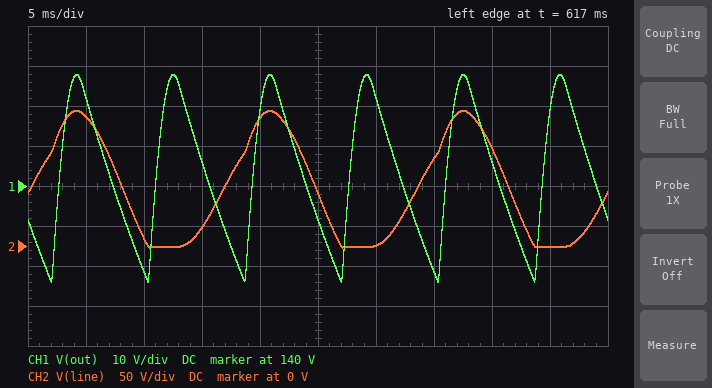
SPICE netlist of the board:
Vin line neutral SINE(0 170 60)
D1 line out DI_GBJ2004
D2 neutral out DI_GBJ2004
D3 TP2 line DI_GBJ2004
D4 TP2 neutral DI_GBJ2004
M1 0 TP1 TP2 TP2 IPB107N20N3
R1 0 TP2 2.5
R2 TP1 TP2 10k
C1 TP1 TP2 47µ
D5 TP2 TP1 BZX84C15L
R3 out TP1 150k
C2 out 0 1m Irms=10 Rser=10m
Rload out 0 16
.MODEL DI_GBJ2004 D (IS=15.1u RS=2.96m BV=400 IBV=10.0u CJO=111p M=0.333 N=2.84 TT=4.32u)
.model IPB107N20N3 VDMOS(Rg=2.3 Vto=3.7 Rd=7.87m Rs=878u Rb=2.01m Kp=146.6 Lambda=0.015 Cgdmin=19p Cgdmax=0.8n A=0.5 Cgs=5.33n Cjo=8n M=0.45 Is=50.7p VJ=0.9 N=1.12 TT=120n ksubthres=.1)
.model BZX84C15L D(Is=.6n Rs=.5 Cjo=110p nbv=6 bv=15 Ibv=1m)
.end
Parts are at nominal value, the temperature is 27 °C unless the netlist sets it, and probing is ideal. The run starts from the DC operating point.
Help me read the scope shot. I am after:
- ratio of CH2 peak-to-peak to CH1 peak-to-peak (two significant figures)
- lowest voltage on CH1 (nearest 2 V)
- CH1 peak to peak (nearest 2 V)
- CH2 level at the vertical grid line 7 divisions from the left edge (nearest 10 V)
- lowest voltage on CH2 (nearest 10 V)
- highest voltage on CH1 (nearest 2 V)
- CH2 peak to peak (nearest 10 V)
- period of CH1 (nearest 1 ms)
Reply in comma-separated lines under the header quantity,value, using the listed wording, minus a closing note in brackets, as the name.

quantity,value
ratio of CH2 peak-to-peak to CH1 peak-to-peak,3.3
lowest voltage on CH1,116 V
CH1 peak to peak,52 V
CH2 level at the vertical grid line 7 divisions from the left edge,110 V
lowest voltage on CH2,0 V
highest voltage on CH1,168 V
CH2 peak to peak,170 V
period of CH1,8 ms
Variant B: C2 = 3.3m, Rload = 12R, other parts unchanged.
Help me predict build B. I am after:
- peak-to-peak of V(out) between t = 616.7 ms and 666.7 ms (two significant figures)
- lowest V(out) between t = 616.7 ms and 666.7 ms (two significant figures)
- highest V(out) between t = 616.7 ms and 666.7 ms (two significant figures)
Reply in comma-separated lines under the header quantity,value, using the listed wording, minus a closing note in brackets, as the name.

quantity,value
peak-to-peak of V(out) between t = 616.7 ms and 666.7 ms,26 V
lowest V(out) between t = 616.7 ms and 666.7 ms,140 V
highest V(out) between t = 616.7 ms and 666.7 ms,170 V
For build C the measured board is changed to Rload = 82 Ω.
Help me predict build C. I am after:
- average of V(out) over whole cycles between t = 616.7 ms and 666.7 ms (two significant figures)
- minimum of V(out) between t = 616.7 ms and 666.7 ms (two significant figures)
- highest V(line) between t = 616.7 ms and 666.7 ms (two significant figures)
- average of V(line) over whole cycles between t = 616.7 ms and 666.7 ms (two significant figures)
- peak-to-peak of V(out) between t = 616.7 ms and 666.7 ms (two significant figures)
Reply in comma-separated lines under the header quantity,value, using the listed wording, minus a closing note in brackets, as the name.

quantity,value
average of V(out) over whole cycles between t = 616.7 ms and 666.7 ms,160 V
minimum of V(out) between t = 616.7 ms and 666.7 ms,150 V
highest V(line) between t = 616.7 ms and 666.7 ms,170 V
average of V(line) over whole cycles between t = 616.7 ms and 666.7 ms,81 V
peak-to-peak of V(out) between t = 616.7 ms and 666.7 ms,14 V
